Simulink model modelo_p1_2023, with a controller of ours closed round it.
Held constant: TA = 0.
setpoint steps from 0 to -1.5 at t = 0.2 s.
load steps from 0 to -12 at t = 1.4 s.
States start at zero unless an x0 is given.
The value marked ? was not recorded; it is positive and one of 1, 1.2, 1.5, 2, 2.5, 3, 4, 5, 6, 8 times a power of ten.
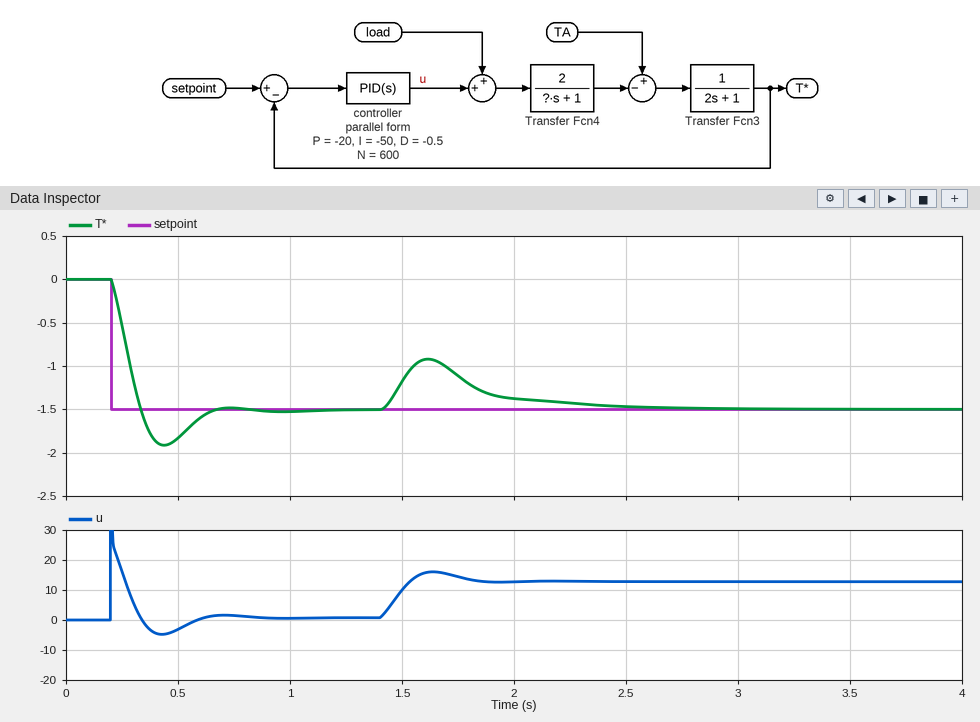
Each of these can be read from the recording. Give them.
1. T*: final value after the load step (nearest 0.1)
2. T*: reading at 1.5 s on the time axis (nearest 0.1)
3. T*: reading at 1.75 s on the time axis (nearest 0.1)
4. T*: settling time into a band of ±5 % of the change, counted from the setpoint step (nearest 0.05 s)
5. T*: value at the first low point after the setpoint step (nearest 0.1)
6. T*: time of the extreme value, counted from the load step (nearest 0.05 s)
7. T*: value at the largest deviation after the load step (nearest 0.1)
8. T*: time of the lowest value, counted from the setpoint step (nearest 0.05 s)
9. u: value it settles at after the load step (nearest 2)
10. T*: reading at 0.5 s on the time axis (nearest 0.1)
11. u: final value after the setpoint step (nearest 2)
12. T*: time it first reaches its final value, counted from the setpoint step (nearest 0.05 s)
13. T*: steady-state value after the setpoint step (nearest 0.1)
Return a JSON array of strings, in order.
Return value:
["-1.5", "-1.2", "-1.1", "0.40 s", "-1.9", "0.20 s", "-0.9", "0.25 s", "12", "-1.8", "0", "0.15 s", "-1.5"]
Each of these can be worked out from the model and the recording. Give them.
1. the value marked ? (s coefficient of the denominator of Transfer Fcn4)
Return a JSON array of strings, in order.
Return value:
["0.1"]
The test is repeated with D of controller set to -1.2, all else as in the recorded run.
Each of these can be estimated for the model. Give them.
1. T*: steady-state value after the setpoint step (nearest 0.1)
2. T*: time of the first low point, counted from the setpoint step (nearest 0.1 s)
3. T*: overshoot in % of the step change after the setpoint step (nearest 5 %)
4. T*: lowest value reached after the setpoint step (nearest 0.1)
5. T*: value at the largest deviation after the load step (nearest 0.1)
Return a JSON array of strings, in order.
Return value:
["-1.5", "0.3 s", "15 %", "-1.7", "-1.0"]
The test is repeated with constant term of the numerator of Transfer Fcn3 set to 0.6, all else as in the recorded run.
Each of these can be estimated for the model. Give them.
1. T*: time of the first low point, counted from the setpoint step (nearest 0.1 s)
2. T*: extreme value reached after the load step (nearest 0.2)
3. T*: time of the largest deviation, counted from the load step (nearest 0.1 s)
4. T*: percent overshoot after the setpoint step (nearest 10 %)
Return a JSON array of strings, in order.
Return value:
["0.3 s", "-1.0", "0.3 s", "30 %"]
